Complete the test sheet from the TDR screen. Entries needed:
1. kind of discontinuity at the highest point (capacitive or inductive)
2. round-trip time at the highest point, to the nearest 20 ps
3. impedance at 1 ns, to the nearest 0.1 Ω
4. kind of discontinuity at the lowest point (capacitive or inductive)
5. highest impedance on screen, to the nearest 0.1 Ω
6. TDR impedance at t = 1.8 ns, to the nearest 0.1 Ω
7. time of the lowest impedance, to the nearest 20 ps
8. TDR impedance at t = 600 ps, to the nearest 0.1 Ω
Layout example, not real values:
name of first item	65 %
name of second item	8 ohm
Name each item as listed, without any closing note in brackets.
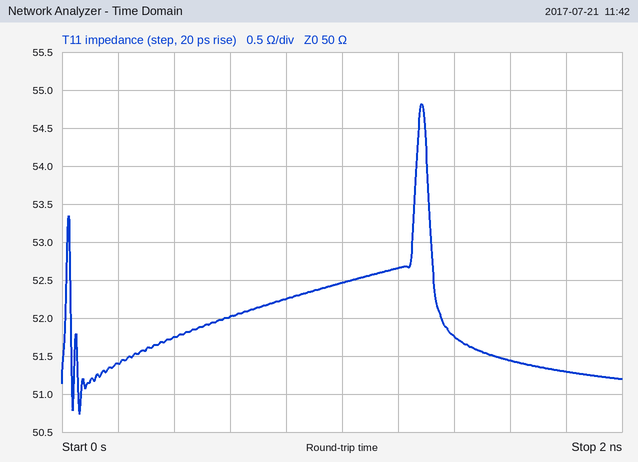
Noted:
kind of discontinuity at the highest point	inductive
round-trip time at the highest point, to the nearest 20 ps	1.28 ns
impedance at 1 ns, to the nearest 0.1 Ω	52.5 Ω
kind of discontinuity at the lowest point	capacitive
highest impedance on screen, to the nearest 0.1 Ω	54.8 Ω
TDR impedance at t = 1.8 ns, to the nearest 0.1 Ω	51.3 Ω
time of the lowest impedance, to the nearest 20 ps	60 ps
TDR impedance at t = 600 ps, to the nearest 0.1 Ω	52.0 Ω
